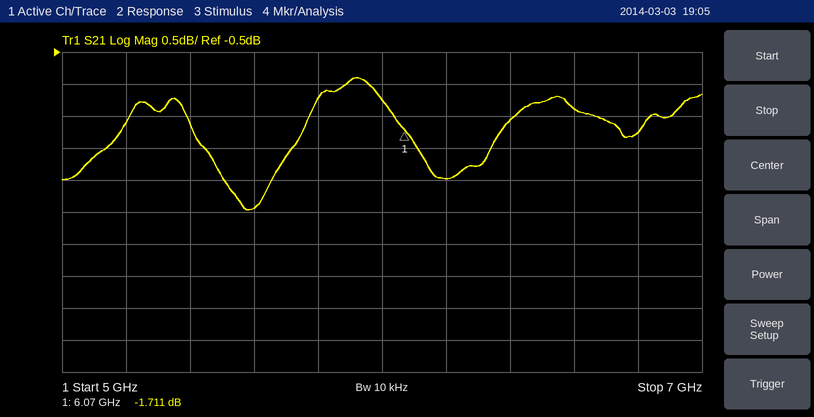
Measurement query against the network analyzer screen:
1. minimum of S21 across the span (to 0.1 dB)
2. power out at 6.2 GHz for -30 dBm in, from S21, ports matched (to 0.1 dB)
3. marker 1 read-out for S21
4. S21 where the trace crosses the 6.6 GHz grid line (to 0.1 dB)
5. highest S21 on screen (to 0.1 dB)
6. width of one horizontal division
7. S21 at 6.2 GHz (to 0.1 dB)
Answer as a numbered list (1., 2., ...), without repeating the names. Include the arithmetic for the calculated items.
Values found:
1. -3.0 dB
2. -30 dBm + (-2.5 dB) = -32.5 dBm
3. -1.711 dB
4. -1.4 dB
5. -0.9 dB
6. 200 MHz
7. -2.5 dB
